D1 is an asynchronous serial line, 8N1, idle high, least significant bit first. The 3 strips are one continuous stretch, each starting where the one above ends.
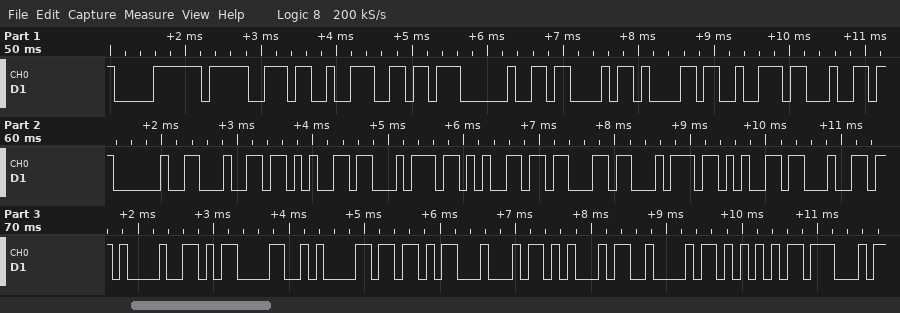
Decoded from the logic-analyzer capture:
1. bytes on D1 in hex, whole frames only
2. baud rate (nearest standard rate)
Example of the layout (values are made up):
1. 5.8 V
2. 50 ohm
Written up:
1. F0 9F 93 B6 20 43 61 72 64 20 64 65 74 65 63 74 65 64 21 0D 0A 5B 44 45 42 55 47
2. 9600 baud
